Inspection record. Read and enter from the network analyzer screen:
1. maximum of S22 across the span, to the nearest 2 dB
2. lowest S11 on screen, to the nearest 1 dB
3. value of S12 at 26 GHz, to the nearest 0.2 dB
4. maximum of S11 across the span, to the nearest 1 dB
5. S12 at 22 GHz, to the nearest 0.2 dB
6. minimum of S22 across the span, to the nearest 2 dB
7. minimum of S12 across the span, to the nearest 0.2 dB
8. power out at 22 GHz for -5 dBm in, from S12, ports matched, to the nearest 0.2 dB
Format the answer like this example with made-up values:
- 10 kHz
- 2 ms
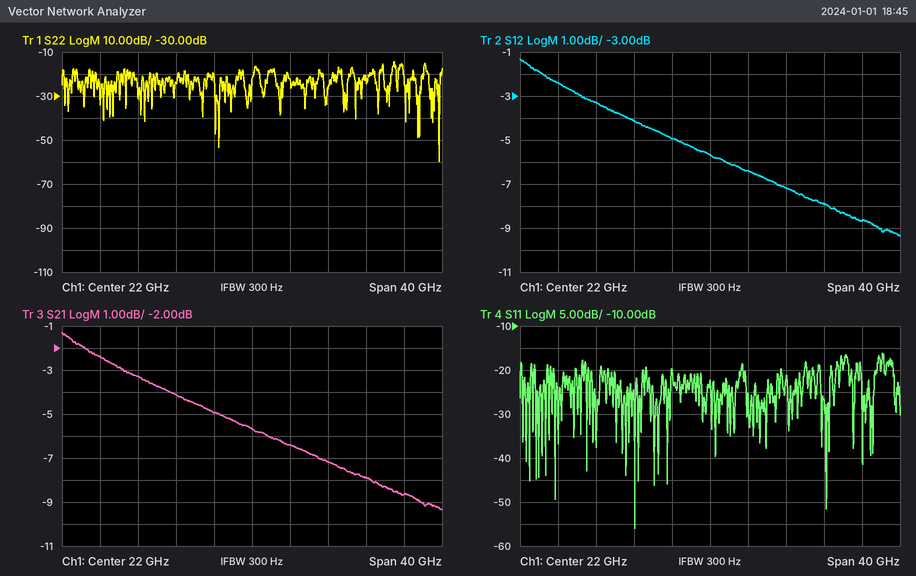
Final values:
- -14 dB
- -56 dB
- -6.4 dB
- -16 dB
- -5.6 dB
- -60 dB
- -9.4 dB
- -10.6 dBm
